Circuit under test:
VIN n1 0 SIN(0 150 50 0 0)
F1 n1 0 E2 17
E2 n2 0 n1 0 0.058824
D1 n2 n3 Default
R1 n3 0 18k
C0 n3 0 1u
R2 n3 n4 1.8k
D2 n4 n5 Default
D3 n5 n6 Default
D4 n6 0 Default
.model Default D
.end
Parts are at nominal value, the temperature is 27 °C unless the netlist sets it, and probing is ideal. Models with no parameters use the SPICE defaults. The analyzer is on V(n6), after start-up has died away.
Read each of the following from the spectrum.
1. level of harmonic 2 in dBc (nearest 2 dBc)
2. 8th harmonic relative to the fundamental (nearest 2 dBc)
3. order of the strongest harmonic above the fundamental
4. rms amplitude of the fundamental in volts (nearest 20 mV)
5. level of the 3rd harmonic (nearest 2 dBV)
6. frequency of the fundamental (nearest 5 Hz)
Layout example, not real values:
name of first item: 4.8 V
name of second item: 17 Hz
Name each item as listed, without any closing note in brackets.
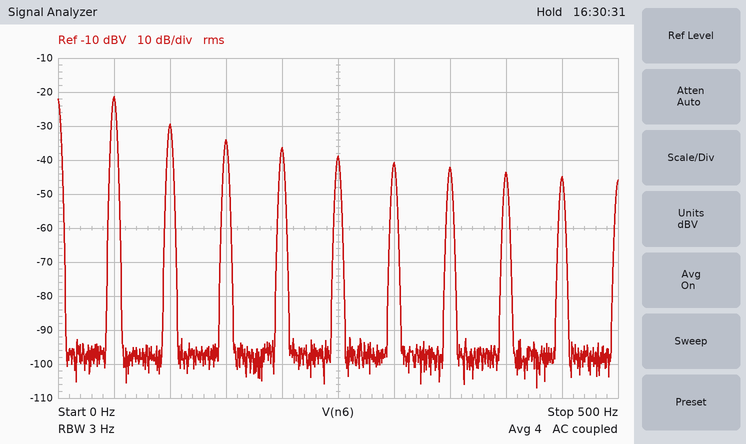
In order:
level of harmonic 2 in dBc: -8 dBc
8th harmonic relative to the fundamental: -22 dBc
order of the strongest harmonic above the fundamental: 2
rms amplitude of the fundamental in volts: 80 mV
level of the 3rd harmonic: -34 dBV
frequency of the fundamental: 50 Hz
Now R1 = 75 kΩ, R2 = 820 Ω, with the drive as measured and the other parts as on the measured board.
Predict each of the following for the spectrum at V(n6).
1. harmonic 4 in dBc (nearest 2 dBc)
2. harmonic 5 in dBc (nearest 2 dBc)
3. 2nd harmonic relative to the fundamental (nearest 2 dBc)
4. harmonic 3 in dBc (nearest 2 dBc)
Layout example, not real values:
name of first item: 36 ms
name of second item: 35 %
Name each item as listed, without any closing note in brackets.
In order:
harmonic 4 in dBc: -16 dBc
harmonic 5 in dBc: -20 dBc
2nd harmonic relative to the fundamental: -10 dBc
harmonic 3 in dBc: -14 dBc
